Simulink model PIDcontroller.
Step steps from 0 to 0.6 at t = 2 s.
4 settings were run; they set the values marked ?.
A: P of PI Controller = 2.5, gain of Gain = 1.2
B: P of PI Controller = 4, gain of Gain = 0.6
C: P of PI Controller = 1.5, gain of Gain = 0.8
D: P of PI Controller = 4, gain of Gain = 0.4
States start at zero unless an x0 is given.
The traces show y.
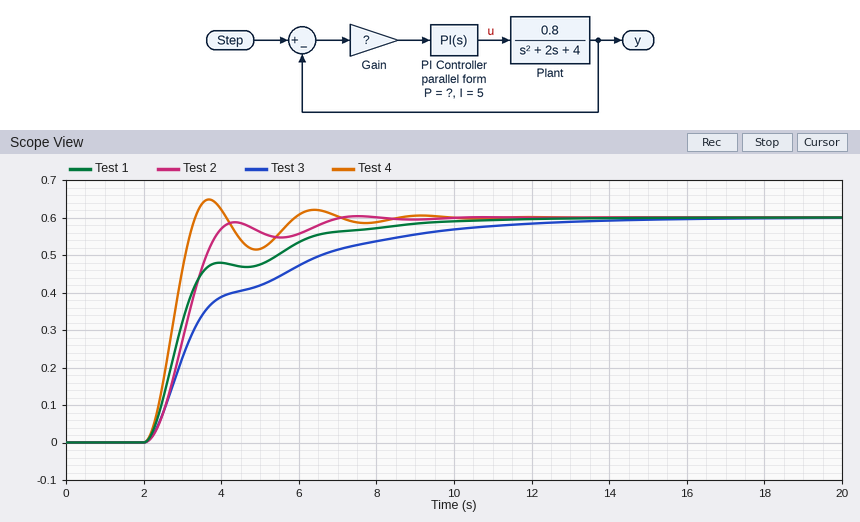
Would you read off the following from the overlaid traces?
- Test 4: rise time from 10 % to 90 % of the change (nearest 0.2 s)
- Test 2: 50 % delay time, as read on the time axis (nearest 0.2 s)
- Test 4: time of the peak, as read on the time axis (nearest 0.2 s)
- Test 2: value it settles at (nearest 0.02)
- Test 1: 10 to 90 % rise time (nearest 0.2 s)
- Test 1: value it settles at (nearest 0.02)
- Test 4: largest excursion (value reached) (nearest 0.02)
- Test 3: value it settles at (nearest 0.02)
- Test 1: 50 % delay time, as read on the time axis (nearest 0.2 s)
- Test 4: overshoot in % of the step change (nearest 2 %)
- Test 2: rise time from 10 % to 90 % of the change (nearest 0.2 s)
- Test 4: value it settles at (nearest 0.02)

0.8 s
3.0 s
3.6 s
0.60
3.8 s
0.60
0.64
0.60
3.0 s
8 %
1.4 s
0.60
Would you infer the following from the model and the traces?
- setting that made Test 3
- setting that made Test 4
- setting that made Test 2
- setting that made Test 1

D
A
C
B
